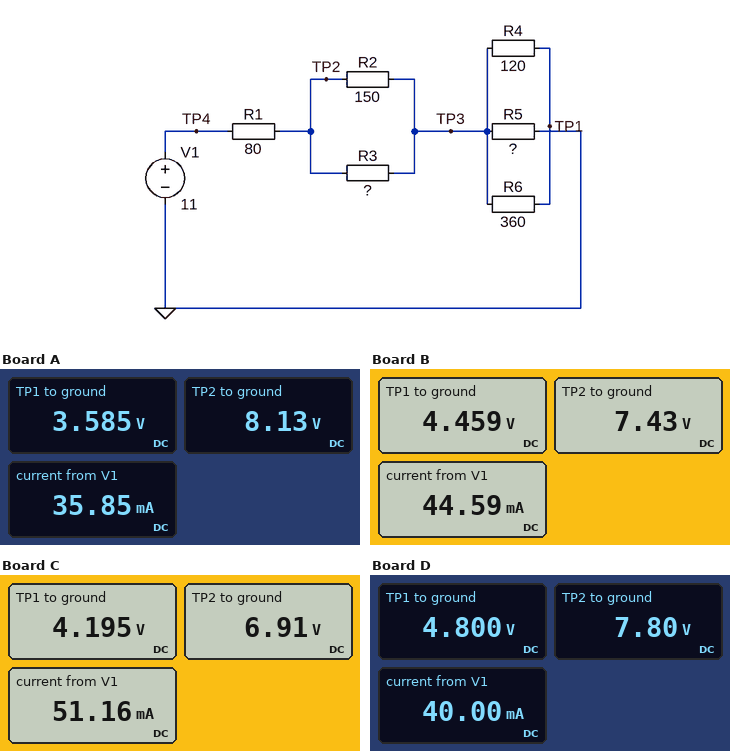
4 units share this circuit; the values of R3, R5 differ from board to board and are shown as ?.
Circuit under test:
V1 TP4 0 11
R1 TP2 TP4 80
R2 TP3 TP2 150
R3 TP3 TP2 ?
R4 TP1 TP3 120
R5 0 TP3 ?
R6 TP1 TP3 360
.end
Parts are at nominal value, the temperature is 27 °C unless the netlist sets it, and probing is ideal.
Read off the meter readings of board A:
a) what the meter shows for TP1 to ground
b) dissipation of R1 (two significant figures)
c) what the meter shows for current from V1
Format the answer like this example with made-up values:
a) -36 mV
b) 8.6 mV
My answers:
a) 3.585 V
b) 100 mW
c) 35.85 mA
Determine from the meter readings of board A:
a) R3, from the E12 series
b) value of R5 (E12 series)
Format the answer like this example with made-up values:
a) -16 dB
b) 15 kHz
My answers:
a) 820 Ω
b) 100 Ω
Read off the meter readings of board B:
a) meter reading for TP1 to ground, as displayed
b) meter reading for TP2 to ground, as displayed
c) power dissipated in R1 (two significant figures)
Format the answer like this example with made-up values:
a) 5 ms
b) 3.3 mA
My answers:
a) 4.459 V
b) 7.43 V
c) 160 mW
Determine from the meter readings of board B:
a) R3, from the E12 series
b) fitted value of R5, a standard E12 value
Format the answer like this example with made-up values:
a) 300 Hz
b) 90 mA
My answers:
a) 120 Ω
b) 100 Ω
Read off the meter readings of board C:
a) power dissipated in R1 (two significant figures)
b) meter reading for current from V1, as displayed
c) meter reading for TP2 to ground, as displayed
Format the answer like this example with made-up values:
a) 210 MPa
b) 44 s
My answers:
a) 210 mW
b) 51.16 mA
c) 6.91 V
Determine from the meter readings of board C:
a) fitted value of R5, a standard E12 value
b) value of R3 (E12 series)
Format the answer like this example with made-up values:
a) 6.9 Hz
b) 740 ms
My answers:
a) 82 Ω
b) 82 Ω
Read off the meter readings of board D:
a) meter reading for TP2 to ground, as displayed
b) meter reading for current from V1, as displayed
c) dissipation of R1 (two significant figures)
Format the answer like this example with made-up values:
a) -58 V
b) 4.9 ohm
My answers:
a) 7.80 V
b) 40.00 mA
c) 130 mW
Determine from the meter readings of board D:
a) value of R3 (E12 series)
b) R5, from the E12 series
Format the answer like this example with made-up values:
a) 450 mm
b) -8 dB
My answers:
a) 150 Ω
b) 120 Ω
